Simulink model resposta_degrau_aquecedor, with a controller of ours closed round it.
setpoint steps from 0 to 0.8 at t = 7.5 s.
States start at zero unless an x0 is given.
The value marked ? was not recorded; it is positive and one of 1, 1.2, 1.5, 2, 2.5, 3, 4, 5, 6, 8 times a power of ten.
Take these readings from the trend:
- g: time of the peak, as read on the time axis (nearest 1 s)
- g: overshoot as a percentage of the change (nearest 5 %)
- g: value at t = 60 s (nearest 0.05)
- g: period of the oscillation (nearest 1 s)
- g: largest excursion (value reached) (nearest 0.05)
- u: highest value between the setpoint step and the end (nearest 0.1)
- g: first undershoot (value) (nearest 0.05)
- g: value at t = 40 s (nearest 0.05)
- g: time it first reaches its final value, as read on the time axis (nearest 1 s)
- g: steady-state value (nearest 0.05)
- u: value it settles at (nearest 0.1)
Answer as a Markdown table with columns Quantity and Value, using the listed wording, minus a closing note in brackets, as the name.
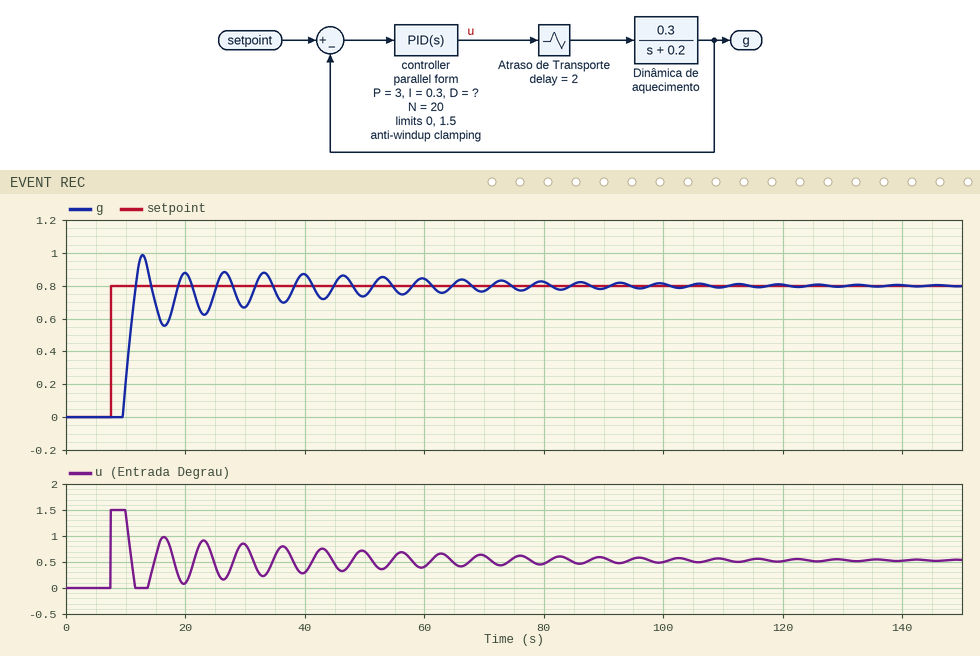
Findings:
| Quantity | Value |
|---|---|
| g: time of the peak, as read on the time axis | 13 s |
| g: overshoot as a percentage of the change | 25 % |
| g: value at t = 60 s | 0.85 |
| g: period of the oscillation | 7 s |
| g: largest excursion (value reached) | 1.00 |
| u: highest value between the setpoint step and the end | 1.5 |
| g: first undershoot (value) | 0.55 |
| g: value at t = 40 s | 0.85 |
| g: time it first reaches its final value, as read on the time axis | 12 s |
| g: steady-state value | 0.80 |
| u: value it settles at | 0.5 |
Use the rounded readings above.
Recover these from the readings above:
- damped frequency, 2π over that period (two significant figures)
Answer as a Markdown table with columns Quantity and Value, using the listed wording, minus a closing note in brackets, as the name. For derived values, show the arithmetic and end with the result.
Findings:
| Quantity | Value |
|---|---|
| damped frequency, 2π over that period | 2π / 7 = 0.90 rad/s |
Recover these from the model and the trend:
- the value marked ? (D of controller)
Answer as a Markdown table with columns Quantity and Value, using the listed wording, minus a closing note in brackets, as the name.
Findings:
| Quantity | Value |
|---|---|
| the value marked ? | 0.8 |
